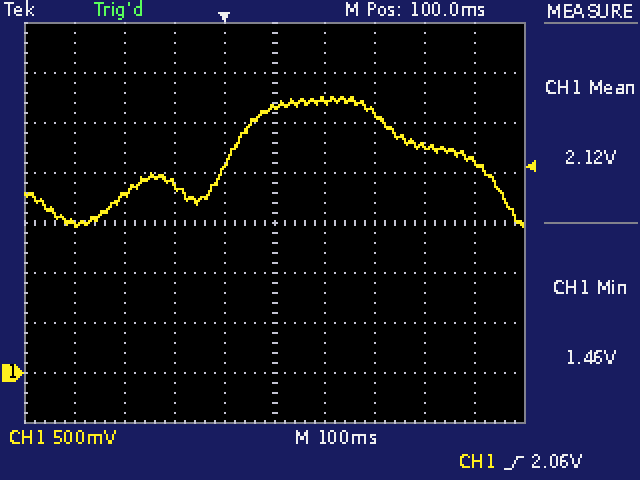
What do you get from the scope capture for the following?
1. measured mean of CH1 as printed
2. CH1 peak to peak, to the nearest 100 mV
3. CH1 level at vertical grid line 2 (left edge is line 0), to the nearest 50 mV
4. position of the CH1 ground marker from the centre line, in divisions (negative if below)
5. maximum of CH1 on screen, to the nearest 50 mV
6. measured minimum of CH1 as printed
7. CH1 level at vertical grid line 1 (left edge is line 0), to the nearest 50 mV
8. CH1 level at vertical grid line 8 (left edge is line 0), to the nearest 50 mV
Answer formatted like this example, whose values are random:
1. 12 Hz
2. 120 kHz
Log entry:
1. 2.12 V
2. 1.30 V
3. 1.80 V
4. -3.0 div
5. 2.75 V
6. 1.46 V
7. 1.50 V
8. 2.25 V
